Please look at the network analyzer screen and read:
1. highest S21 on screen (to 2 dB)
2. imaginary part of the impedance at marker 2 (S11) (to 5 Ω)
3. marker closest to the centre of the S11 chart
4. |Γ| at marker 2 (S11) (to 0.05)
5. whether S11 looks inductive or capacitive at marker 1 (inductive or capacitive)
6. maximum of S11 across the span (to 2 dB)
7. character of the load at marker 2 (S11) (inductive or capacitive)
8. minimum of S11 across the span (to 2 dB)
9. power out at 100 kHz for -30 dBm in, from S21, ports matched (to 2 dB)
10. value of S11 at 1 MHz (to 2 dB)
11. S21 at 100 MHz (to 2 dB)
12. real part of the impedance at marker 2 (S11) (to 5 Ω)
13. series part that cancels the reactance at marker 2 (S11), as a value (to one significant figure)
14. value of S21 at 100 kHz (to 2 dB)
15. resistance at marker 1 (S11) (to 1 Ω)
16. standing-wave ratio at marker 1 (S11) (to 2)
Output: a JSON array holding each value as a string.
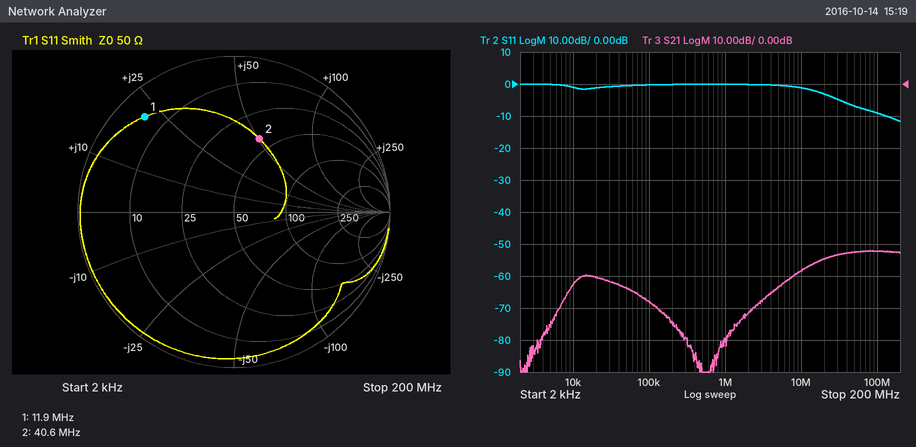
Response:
["-52 dB", "+50 Ω", "marker 2", "0.50", "inductive", "0 dB", "inductive", "-12 dB", "-98 dBm", "0 dB", "-52 dB", "40 Ω", "80 pF", "-68 dB", "5 Ω", "12"]
